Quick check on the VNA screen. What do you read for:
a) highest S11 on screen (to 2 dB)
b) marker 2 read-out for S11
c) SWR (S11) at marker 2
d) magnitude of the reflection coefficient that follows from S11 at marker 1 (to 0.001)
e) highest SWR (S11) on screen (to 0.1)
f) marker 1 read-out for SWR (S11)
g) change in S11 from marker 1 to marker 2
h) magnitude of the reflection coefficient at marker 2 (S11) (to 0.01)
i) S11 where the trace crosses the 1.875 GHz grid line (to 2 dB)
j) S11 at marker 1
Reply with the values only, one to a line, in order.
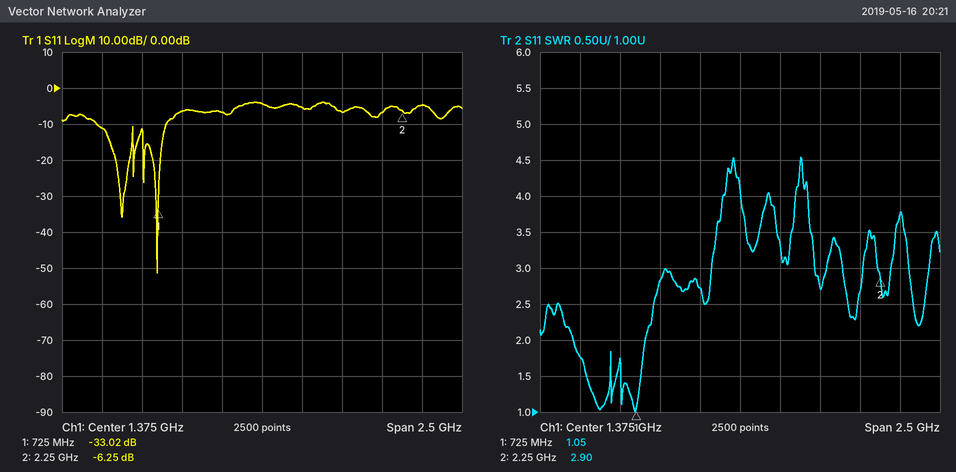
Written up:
-4 dB
-6.25 dB
2.90
0.022
4.5
1.05
26.77 dB
0.49
-6 dB
-33.02 dB
